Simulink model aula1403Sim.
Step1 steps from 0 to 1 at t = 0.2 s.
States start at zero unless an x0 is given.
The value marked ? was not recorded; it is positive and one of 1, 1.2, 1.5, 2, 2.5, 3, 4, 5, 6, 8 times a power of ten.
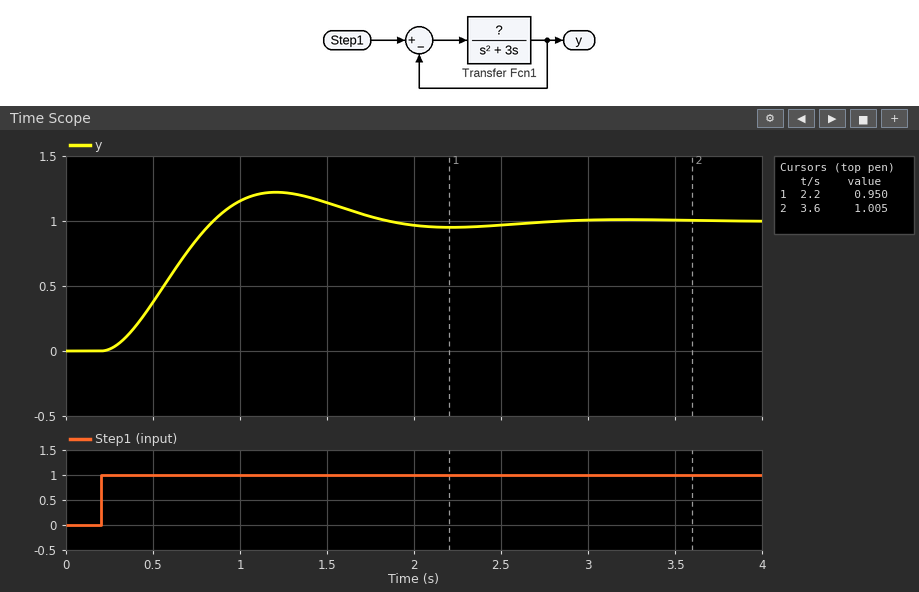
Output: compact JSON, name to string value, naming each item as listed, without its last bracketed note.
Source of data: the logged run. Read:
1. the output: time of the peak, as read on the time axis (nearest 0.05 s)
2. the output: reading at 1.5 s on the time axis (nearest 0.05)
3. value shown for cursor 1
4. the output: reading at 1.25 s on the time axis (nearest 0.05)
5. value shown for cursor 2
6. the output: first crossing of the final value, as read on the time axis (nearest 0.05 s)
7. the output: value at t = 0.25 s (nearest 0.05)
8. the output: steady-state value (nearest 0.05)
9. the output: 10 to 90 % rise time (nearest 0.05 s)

{"the output: time of the peak, as read on the time axis": "1.20 s", "the output: reading at 1.5 s on the time axis": "1.15", "value shown for cursor 1": "0.950", "the output: reading at 1.25 s on the time axis": "1.20", "value shown for cursor 2": "1.005", "the output: first crossing of the final value, as read on the time axis": "0.85 s", "the output: value at t = 0.25 s": "0.00", "the output: steady-state value": "1.00", "the output: 10 to 90 % rise time": "0.45 s"}
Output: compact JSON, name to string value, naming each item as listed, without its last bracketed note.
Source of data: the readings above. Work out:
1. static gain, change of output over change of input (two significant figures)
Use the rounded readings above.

{"static gain, change of output over change of input": "1.0"}
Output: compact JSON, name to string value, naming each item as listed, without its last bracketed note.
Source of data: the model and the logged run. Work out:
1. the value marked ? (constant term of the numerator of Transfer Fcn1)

{"the value marked ?": "12"}
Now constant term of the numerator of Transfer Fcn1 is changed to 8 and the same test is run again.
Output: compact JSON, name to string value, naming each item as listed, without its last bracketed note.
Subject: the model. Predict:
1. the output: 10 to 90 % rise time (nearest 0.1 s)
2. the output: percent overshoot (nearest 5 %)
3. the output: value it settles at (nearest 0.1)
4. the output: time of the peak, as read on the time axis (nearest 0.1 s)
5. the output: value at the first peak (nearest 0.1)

{"the output: 10 to 90 % rise time": "0.6 s", "the output: percent overshoot": "15 %", "the output: value it settles at": "1.0", "the output: time of the peak, as read on the time axis": "1.5 s", "the output: value at the first peak": "1.1"}
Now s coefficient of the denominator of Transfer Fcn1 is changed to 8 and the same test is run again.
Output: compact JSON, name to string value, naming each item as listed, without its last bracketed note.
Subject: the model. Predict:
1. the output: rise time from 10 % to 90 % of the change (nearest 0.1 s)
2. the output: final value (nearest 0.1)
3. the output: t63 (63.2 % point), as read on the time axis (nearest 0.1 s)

{"the output: rise time from 10 % to 90 % of the change": "1.2 s", "the output: final value": "1.0", "the output: t63 (63.2 % point), as read on the time axis": "0.9 s"}
